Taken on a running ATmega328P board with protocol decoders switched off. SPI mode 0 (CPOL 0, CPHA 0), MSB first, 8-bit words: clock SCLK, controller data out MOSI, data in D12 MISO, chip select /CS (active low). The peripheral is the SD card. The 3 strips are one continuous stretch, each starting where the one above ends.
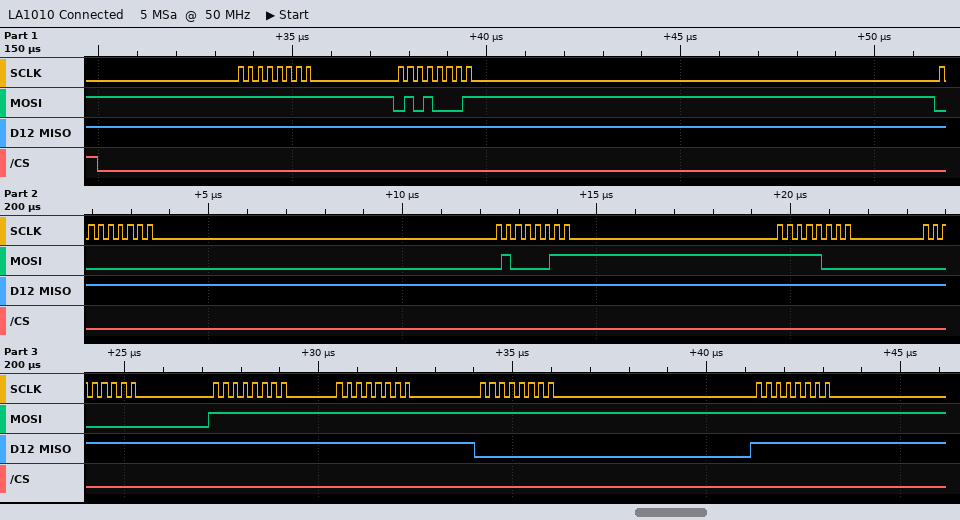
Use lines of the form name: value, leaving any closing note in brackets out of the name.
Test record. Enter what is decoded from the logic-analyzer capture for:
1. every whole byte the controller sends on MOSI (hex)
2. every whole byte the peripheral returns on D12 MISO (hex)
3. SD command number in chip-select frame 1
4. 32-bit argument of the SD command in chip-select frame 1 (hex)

every whole byte the controller sends on MOSI: FF 51 00 43 F8 00 FF FF FF FF
every whole byte the peripheral returns on D12 MISO: FF FF FF FF FF FF FF FF 00 FF
SD command number in chip-select frame 1: CMD17
32-bit argument of the SD command in chip-select frame 1: 0x0043F800
